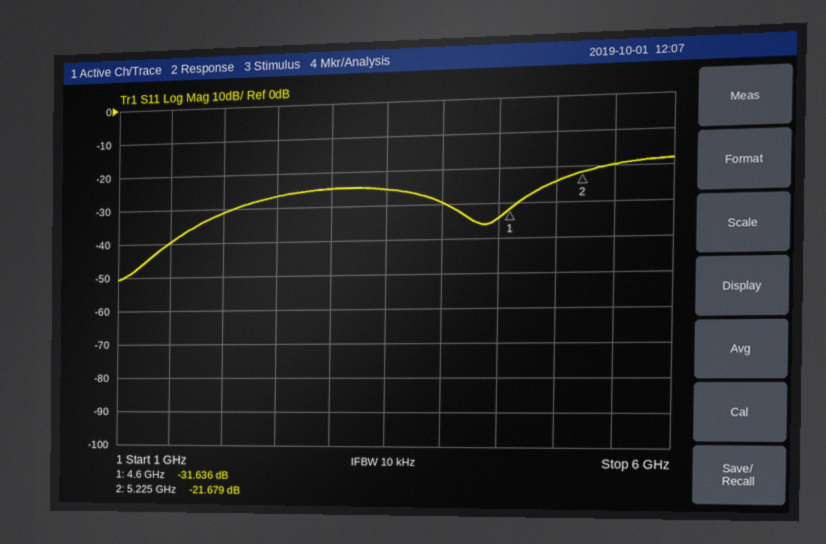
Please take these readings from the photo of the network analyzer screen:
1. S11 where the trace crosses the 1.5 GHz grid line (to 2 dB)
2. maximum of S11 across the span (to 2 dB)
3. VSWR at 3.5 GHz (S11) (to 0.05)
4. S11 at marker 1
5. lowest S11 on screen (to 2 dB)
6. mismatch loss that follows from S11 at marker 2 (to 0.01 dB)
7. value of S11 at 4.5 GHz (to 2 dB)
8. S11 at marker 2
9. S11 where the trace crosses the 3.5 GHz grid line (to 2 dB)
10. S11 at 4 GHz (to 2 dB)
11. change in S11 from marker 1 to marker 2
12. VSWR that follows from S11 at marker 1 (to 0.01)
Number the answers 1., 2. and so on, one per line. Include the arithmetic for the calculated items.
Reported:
1. -40 dB
2. -18 dB
3. |Γ| = 10^(-26/20) = 0.0501; VSWR = (1 + 0.0501)/(1 − 0.0501) ≈ 1.11, so 1.10 to the nearest 0.05
4. -31.636 dB
5. -50 dB
6. −10 log10(1 − 10^(-21.679/10)) ≈ 0.03 dB
7. -34 dB
8. -21.679 dB
9. -26 dB
10. -30 dB
11. -21.679 − (-31.636) = 9.957 dB
12. (1 + 0.0262)/(1 − 0.0262) ≈ 1.05
